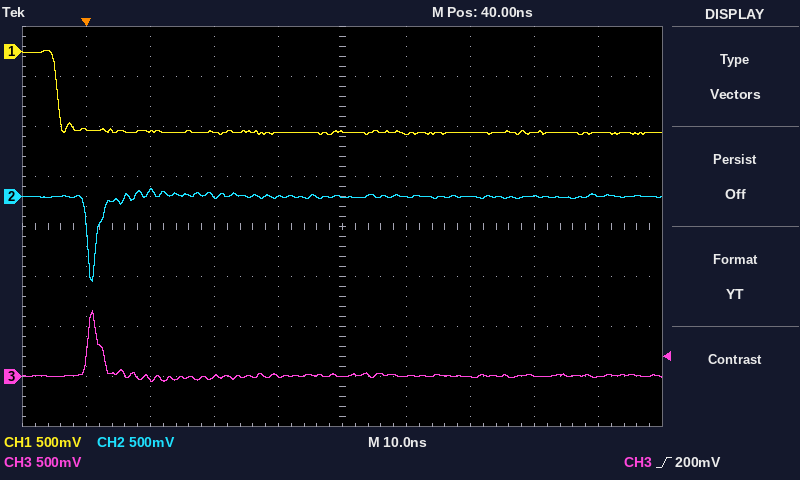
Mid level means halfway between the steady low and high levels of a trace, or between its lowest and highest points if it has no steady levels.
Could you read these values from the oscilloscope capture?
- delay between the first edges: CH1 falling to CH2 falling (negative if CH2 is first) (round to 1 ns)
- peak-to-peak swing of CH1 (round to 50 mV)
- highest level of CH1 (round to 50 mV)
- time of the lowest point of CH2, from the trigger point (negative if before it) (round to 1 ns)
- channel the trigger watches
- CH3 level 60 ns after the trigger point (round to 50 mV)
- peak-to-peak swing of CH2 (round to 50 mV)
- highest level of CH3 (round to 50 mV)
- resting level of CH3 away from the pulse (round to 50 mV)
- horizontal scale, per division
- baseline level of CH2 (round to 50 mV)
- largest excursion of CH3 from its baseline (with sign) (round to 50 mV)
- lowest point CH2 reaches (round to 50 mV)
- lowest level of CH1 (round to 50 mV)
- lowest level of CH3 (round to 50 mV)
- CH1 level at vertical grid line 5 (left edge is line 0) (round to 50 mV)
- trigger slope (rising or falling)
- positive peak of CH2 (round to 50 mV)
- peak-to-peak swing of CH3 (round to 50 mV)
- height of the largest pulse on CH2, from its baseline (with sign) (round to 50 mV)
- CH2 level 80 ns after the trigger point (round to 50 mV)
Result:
+5 ns
850 mV
0 mV
+1 ns
CH3
0 mV
950 mV
650 mV
0 mV
10 ns
0 mV
+650 mV
-850 mV
-850 mV
-50 mV
-800 mV
rising
100 mV
700 mV
-850 mV
0 mV
